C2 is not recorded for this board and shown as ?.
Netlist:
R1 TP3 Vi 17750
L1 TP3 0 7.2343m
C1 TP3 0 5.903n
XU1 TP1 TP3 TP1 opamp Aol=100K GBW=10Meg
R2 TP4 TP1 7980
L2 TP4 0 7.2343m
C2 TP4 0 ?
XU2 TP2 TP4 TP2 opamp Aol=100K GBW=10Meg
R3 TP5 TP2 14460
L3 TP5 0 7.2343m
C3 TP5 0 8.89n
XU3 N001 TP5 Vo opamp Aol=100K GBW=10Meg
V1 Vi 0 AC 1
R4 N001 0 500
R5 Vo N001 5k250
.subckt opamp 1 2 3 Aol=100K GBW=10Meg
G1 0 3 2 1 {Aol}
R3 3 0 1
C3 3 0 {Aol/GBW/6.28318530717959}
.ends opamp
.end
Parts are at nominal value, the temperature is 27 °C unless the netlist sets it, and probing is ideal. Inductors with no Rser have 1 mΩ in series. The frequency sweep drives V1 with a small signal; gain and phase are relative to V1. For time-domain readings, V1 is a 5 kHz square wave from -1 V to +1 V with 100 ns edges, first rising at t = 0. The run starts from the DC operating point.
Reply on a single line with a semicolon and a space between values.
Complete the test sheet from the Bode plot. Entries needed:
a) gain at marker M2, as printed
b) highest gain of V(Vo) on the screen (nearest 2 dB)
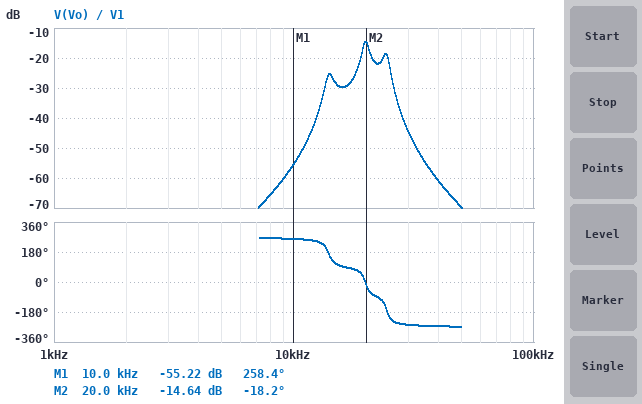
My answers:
-14.64 dB; -14 dB
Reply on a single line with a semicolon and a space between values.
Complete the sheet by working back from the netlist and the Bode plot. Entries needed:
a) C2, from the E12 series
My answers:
18 nF
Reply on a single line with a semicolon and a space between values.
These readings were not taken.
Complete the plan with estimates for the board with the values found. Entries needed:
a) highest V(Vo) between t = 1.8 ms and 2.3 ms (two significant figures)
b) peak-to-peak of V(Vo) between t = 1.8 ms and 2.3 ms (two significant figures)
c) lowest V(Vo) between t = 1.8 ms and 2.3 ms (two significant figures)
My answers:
34 mV; 68 mV; -34 mV
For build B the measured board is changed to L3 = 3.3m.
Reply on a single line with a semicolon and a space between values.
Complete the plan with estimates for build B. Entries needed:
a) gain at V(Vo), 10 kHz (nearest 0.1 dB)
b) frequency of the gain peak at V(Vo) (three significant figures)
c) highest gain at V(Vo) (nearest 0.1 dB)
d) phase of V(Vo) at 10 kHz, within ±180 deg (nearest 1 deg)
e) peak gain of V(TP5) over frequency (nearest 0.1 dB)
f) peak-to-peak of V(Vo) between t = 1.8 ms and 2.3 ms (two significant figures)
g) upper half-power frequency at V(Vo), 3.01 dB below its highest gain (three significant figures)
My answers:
-63.5 dB; 29.3 kHz; -20.7 dB; -100 deg; -41.9 dB; 45 mV; 29.9 kHz
